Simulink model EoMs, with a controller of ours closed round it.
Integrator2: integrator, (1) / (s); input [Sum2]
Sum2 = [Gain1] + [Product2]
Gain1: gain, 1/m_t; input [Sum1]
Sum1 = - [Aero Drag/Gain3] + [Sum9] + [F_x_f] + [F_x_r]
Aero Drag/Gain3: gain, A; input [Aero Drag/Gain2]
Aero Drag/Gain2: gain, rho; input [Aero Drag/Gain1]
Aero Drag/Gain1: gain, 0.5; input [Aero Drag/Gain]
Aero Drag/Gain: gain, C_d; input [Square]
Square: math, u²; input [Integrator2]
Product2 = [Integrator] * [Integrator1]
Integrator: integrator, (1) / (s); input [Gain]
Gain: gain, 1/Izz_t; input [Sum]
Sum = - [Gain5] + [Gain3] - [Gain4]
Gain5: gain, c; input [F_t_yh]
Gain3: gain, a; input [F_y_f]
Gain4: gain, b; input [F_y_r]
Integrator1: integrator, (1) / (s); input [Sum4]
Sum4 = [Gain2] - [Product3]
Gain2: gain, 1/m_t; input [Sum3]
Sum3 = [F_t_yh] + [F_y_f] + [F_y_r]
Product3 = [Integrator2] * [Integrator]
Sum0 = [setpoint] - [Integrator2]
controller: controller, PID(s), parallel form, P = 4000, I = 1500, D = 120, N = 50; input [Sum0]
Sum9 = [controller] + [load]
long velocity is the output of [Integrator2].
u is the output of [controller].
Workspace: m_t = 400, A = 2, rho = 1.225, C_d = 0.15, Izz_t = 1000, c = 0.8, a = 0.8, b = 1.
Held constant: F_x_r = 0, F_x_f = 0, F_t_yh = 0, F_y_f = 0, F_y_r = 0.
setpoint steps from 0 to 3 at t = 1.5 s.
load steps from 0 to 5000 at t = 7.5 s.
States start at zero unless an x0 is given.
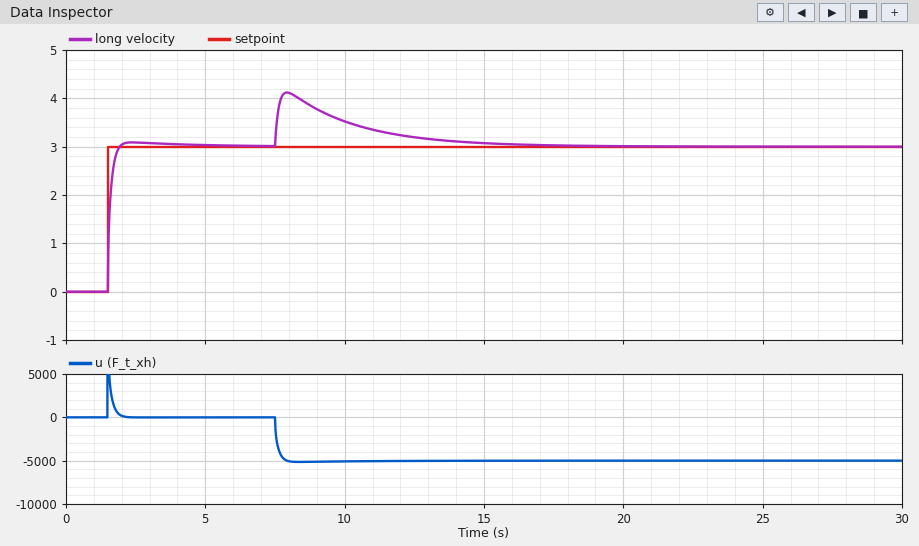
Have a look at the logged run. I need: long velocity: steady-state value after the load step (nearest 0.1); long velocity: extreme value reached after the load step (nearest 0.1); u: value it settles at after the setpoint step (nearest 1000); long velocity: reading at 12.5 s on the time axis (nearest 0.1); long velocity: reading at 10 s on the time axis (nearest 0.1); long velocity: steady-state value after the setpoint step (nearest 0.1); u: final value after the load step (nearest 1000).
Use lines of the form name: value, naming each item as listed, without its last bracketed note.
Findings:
long velocity: steady-state value after the load step: 3.0
long velocity: extreme value reached after the load step: 4.1
u: value it settles at after the setpoint step: 0
long velocity: reading at 12.5 s on the time axis: 3.2
long velocity: reading at 10 s on the time axis: 3.5
long velocity: steady-state value after the setpoint step: 3.0
u: final value after the load step: -5000
